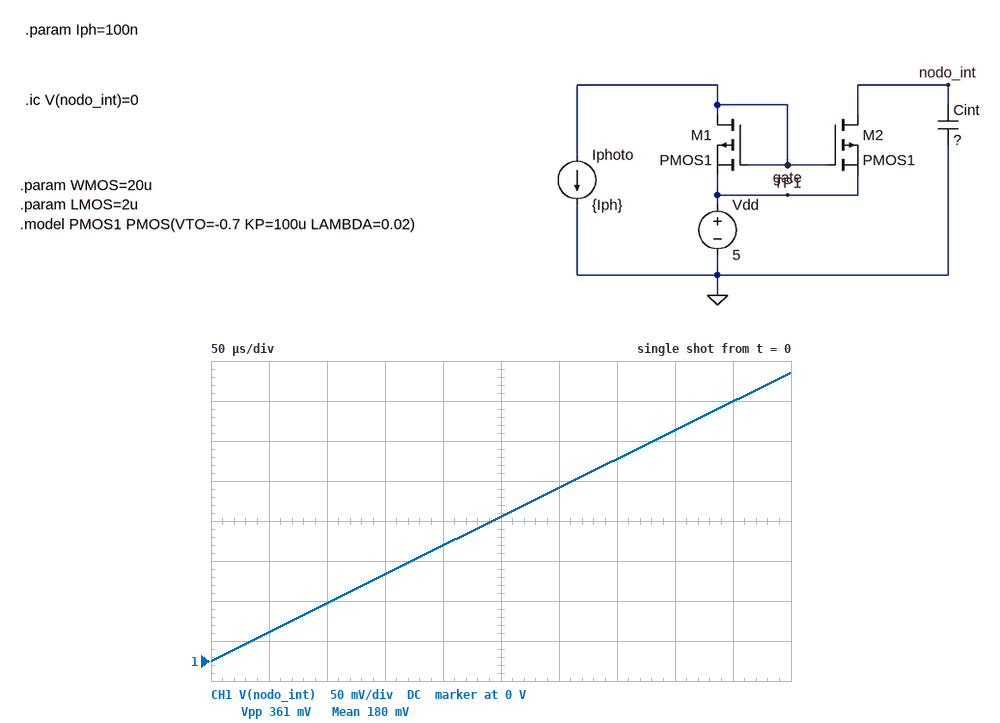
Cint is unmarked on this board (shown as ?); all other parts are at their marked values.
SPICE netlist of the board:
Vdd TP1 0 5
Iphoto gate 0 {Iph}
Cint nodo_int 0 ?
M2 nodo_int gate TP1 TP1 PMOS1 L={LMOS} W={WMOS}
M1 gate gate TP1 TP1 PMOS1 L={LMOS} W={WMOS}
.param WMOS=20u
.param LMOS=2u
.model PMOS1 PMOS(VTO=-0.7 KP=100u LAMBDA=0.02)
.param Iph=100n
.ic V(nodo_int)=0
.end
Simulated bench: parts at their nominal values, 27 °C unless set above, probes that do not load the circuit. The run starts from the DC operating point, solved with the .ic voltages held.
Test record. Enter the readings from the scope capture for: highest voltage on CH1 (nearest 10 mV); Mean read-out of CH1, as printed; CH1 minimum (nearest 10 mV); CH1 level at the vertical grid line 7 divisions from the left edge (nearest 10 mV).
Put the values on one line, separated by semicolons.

360 mV; 180 mV; 0 V; 250 mV
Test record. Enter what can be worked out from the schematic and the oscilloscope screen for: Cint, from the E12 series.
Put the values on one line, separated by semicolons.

150 pF
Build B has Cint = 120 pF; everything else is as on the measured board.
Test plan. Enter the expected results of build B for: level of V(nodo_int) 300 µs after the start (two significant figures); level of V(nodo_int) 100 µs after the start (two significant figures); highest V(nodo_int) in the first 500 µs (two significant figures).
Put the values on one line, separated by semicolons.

270 mV; 90 mV; 450 mV
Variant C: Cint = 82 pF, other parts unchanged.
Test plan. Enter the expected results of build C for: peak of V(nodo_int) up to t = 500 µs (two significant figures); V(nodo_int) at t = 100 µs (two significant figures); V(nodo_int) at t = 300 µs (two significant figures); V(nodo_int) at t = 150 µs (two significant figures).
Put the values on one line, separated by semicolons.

660 mV; 130 mV; 400 mV; 200 mV
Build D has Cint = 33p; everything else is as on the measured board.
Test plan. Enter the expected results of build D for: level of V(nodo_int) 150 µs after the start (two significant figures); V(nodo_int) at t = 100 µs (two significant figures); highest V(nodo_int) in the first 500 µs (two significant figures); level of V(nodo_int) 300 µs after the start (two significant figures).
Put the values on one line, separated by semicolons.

490 mV; 330 mV; 1.6 V; 980 mV
